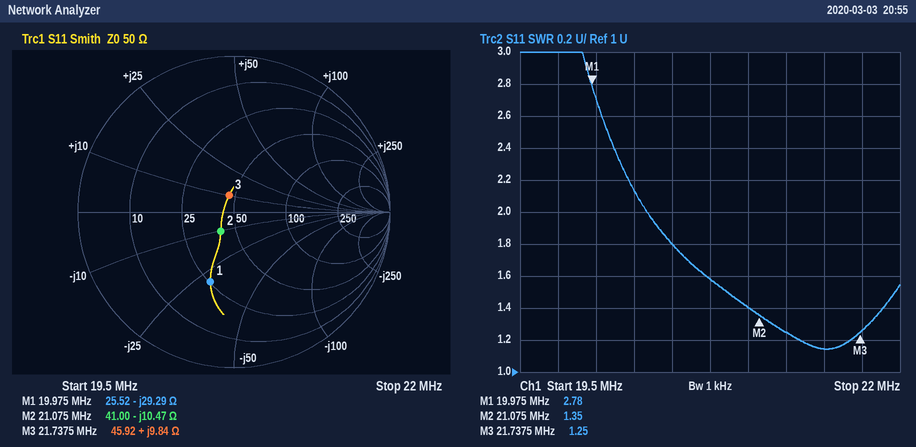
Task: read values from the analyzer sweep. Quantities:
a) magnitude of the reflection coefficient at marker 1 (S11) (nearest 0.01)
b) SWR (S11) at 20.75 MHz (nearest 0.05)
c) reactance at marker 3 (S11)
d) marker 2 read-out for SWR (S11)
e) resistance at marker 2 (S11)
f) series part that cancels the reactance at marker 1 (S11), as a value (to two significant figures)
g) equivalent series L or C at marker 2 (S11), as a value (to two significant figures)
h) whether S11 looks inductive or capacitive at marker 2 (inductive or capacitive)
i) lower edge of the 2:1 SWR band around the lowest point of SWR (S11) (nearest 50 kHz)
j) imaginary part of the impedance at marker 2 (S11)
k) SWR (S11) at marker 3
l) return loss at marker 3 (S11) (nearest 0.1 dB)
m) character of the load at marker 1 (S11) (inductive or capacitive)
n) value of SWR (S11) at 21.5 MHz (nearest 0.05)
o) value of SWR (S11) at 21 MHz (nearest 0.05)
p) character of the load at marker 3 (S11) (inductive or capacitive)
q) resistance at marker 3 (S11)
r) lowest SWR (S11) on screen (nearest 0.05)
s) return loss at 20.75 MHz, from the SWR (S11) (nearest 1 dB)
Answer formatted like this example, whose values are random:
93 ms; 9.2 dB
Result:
0.47; 1.60; +9.84 Ω; 1.35; 41.00 Ω; 230 nH; 720 pF; capacitive; 20.35 MHz; -10.47 Ω; 1.25; 19.1 dB; capacitive; 1.15; 1.40; inductive; 45.92 Ω; 1.15; 13 dB
